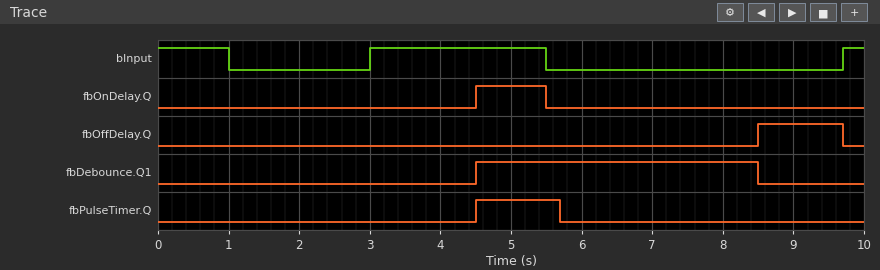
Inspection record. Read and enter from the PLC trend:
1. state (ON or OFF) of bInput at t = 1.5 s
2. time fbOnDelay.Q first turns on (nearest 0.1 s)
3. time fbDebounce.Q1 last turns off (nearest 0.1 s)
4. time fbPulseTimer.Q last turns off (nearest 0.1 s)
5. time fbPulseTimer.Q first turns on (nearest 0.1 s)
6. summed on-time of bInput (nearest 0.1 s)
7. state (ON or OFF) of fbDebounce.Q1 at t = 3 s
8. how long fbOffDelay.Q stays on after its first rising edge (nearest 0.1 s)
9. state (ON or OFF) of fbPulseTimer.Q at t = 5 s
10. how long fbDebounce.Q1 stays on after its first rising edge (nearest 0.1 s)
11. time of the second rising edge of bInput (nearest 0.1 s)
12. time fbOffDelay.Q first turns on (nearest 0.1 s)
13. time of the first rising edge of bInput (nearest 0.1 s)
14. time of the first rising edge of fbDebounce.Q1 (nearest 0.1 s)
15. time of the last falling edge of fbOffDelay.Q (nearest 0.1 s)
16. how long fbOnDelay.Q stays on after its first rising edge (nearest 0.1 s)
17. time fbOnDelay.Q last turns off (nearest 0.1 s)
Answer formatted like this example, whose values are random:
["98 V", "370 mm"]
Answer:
["OFF", "4.5 s", "8.5 s", "5.7 s", "4.5 s", "3.8 s", "OFF", "1.2 s", "ON", "4.0 s", "9.7 s", "8.5 s", "3.0 s", "4.5 s", "9.7 s", "1.0 s", "5.5 s"]
